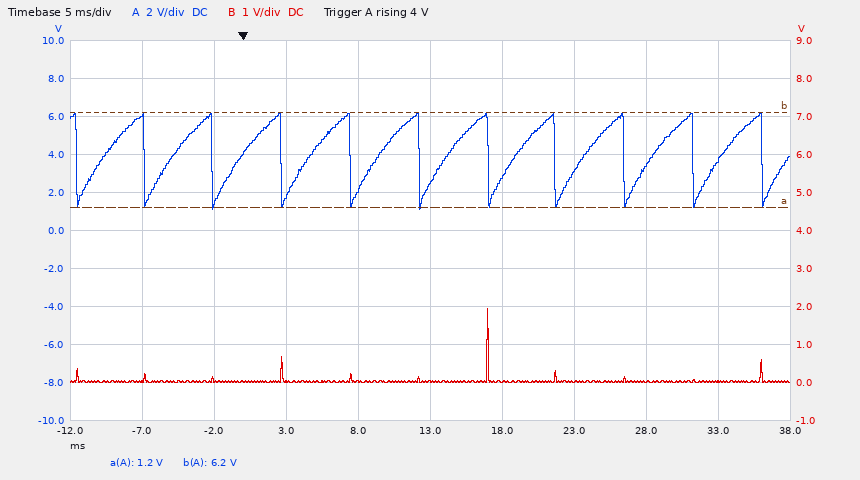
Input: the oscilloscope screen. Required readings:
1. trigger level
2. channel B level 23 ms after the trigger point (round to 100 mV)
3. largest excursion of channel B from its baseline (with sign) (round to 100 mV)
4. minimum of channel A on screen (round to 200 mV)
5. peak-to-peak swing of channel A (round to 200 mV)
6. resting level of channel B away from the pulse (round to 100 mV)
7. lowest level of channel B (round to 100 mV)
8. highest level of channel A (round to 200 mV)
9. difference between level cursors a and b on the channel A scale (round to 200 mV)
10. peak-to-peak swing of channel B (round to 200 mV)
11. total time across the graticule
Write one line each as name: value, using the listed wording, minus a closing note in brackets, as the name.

trigger level: 4 V
channel B level 23 ms after the trigger point: 0.0 V
largest excursion of channel B from its baseline (with sign): +1.9 V
minimum of channel A on screen: 1.2 V
peak-to-peak swing of channel A: 5.0 V
resting level of channel B away from the pulse: 0.0 V
lowest level of channel B: 0.0 V
highest level of channel A: 6.2 V
difference between level cursors a and b on the channel A scale: 5.0 V
peak-to-peak swing of channel B: 2.0 V
total time across the graticule: 50 ms
